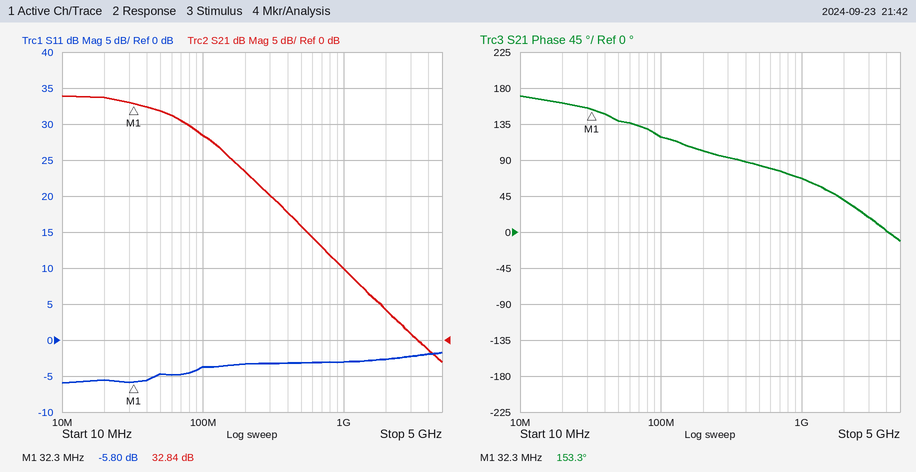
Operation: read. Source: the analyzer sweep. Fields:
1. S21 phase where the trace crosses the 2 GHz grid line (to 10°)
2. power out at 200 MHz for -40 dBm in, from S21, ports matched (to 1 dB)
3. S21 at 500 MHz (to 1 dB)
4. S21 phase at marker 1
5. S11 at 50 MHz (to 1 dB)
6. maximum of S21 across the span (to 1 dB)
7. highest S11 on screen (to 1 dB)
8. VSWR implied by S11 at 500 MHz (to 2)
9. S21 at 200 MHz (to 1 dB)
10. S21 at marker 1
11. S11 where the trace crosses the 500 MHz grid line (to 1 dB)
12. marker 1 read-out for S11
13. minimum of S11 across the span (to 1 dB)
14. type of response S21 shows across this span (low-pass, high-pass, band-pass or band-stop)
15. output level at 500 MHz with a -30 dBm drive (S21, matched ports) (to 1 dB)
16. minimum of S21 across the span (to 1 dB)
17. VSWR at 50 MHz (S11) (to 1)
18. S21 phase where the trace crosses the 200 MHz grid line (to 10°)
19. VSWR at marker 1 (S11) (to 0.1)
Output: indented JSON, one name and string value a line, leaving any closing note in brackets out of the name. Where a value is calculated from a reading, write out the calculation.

{
  "S21 phase where the trace crosses the 2 GHz grid line": "40°",
  "power out at 200 MHz for -40 dBm in, from S21, ports matched": "-40 dBm + (23 dB) = -17 dBm",
  "S21 at 500 MHz": "16 dB",
  "S21 phase at marker 1": "153.3°",
  "S11 at 50 MHz": "-5 dB",
  "maximum of S21 across the span": "34 dB",
  "highest S11 on screen": "-2 dB",
  "VSWR implied by S11 at 500 MHz": "|Γ| = 10^(-3/20) = 0.7079; VSWR = (1 + 0.7079)/(1 − 0.7079) ≈ 6",
  "S21 at 200 MHz": "23 dB",
  "S21 at marker 1": "32.84 dB",
  "S11 where the trace crosses the 500 MHz grid line": "-3 dB",
  "marker 1 read-out for S11": "-5.80 dB",
  "minimum of S11 across the span": "-6 dB",
  "type of response S21 shows across this span": "low-pass",
  "output level at 500 MHz with a -30 dBm drive (S21, matched ports)": "-30 dBm + (16 dB) = -14 dBm",
  "minimum of S21 across the span": "-3 dB",
  "VSWR at 50 MHz (S11)": "|Γ| = 10^(-5/20) = 0.5623; VSWR = (1 + 0.5623)/(1 − 0.5623) ≈ 4",
  "S21 phase where the trace crosses the 200 MHz grid line": "100°",
  "VSWR at marker 1 (S11)": "(1 + 0.5129)/(1 − 0.5129) ≈ 3.1"
}
